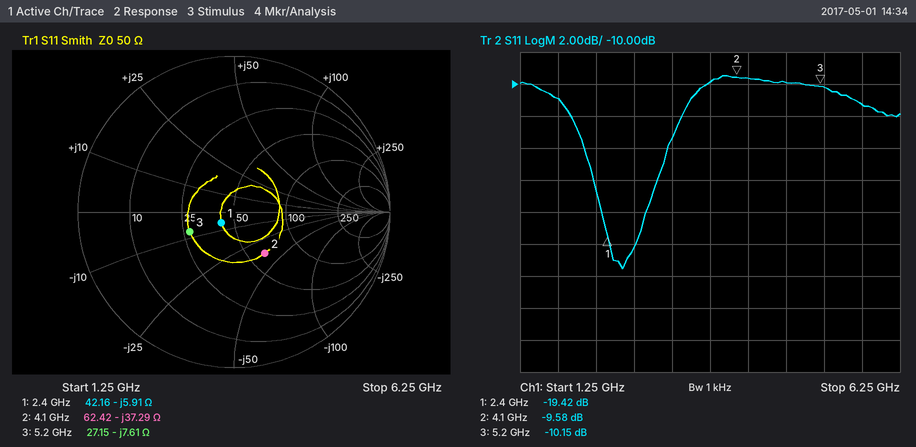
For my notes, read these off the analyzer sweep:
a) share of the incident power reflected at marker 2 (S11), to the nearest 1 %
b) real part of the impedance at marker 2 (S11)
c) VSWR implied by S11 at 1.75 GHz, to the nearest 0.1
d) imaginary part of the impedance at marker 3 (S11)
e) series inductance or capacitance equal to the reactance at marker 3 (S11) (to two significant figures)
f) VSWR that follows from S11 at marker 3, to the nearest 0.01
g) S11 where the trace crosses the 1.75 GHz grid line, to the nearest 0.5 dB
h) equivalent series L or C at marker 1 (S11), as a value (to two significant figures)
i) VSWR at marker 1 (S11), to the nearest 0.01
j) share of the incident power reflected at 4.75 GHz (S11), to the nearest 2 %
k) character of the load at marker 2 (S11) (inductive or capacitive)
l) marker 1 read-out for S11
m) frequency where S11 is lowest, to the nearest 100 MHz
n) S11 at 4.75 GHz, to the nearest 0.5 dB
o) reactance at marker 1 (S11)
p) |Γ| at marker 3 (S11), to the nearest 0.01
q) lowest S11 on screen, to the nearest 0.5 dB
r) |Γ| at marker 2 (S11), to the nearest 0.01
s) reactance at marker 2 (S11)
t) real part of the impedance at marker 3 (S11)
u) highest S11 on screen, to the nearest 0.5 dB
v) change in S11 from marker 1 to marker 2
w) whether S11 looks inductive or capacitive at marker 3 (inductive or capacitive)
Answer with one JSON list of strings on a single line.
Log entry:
["11 %", "62.42 Ω", "1.8", "-7.61 Ω", "4.0 pF", "1.90", "-11.0 dB", "11 pF", "1.24", "10 %", "capacitive", "-19.42 dB", "2.6 GHz", "-10.0 dB", "-5.91 Ω", "0.31", "-21.5 dB", "0.33", "-37.29 Ω", "27.15 Ω", "-9.5 dB", "9.84 dB", "capacitive"]
